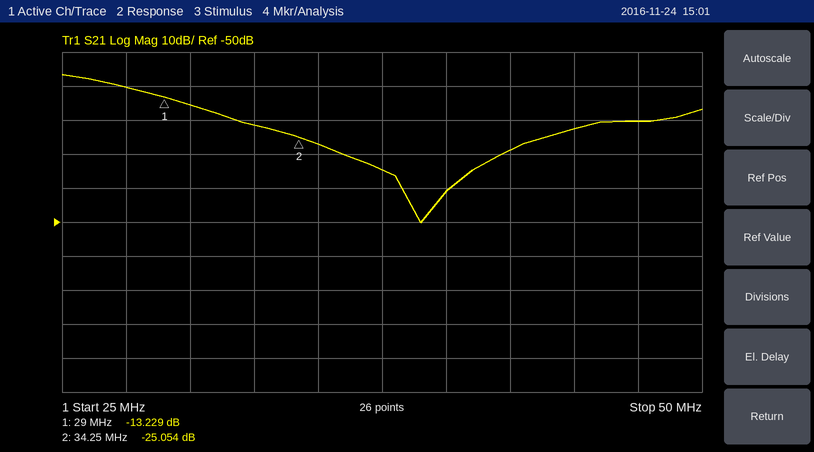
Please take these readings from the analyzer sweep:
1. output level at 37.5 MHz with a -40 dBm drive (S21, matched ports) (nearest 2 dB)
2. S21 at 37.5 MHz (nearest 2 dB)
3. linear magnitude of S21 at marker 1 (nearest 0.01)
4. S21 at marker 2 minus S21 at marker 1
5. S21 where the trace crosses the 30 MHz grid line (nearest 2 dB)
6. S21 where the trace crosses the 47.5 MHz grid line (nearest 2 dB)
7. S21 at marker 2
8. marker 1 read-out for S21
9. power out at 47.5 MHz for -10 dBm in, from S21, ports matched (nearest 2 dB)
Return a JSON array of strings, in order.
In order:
["-74 dBm", "-34 dB", "0.22", "-11.825 dB", "-16 dB", "-20 dB", "-25.054 dB", "-13.229 dB", "-30 dBm"]
